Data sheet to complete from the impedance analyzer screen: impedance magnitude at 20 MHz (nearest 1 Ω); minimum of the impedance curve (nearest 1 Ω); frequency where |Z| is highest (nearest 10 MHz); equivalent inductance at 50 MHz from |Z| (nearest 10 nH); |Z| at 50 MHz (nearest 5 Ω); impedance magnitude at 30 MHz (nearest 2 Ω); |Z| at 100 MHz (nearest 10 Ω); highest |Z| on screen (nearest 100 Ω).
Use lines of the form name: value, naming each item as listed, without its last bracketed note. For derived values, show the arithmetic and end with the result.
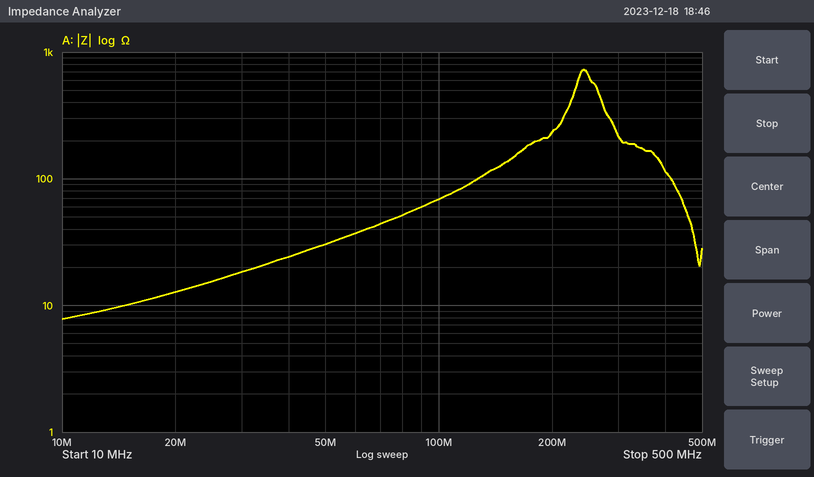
impedance magnitude at 20 MHz: 13 Ω
minimum of the impedance curve: 8 Ω
frequency where |Z| is highest: 240 MHz
equivalent inductance at 50 MHz from |Z|: L = 30 Ω/(2π × 50 MHz) ≈ 95.5 nH, so 100 nH to the nearest 10 nH
|Z| at 50 MHz: 30 Ω
impedance magnitude at 30 MHz: 18 Ω
|Z| at 100 MHz: 70 Ω
highest |Z| on screen: 700 Ω
